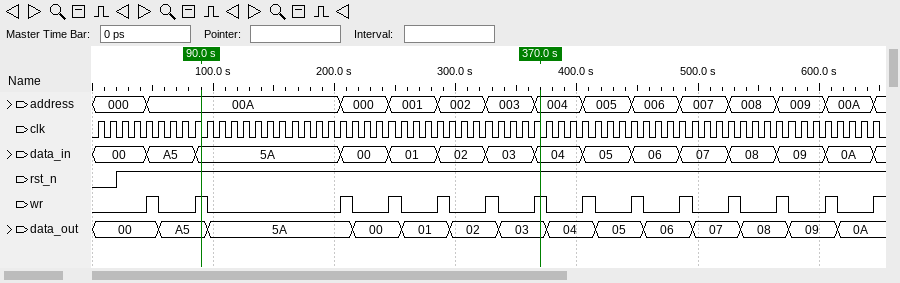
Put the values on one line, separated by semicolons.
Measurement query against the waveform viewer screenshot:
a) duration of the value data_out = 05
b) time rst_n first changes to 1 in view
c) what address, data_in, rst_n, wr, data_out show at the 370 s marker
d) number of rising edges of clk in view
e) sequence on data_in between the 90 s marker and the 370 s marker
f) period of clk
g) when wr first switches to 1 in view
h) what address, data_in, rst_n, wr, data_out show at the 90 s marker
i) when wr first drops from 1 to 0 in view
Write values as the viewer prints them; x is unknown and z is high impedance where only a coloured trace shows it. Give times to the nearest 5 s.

40 s; 20 s; address=004, data_in=04, rst_n=1, wr=1, data_out=03; 65; 5A, 00, 01, 02, 03, 04; 10 s; 45 s; address=00A, data_in=5A, rst_n=1, wr=1, data_out=A5; 55 s
